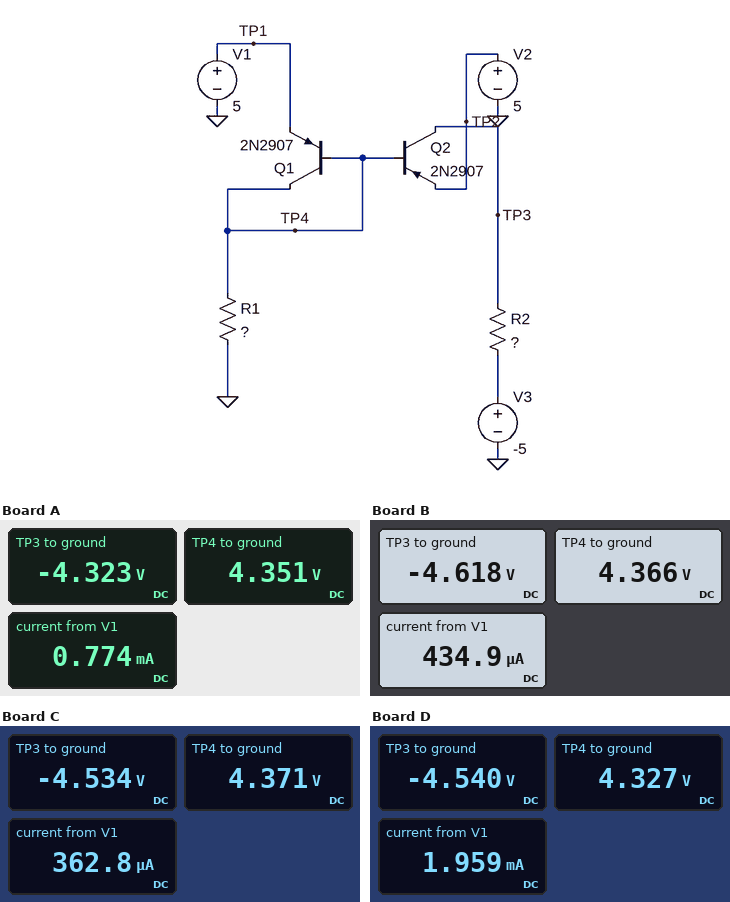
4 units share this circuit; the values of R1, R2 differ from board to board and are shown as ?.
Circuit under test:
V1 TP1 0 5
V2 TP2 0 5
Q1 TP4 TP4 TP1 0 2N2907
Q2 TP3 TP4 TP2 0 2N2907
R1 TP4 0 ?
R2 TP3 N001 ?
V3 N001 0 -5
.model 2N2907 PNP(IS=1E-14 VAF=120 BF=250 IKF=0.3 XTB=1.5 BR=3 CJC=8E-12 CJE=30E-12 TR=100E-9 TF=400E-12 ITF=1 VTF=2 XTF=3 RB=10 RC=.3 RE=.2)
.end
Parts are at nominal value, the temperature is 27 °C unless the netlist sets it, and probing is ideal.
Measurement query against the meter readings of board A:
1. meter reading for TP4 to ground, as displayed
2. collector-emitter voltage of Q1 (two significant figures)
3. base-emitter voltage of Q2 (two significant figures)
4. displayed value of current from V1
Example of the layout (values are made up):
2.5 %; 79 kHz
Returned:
4.351 V; -650 mV; -650 mV; 0.774 mA
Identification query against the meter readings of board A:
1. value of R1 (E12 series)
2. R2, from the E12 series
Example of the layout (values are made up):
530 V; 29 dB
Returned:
5.6 kΩ; 820 Ω
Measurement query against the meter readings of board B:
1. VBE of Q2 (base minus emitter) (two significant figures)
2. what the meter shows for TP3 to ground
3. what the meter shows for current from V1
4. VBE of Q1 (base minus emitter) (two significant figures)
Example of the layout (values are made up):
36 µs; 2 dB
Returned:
-630 mV; -4.618 V; 434.9 µA; -630 mV
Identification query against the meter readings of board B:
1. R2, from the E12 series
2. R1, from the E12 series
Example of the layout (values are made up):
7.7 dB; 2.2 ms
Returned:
820 Ω; 10 kΩ
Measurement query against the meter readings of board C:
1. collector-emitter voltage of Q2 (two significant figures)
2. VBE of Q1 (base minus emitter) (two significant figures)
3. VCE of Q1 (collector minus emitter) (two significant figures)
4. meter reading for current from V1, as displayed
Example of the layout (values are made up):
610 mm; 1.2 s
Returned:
-9.5 V; -630 mV; -630 mV; 362.8 µA
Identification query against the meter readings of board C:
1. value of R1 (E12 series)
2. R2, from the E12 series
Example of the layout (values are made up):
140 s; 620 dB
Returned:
12 kΩ; 1.2 kΩ
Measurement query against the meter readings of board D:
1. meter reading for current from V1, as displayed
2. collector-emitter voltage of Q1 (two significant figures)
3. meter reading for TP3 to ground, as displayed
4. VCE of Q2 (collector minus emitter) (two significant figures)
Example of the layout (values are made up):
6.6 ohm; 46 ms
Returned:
1.959 mA; -670 mV; -4.540 V; -9.5 V
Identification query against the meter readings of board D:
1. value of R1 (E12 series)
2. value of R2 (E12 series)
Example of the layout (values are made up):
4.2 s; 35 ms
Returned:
2.2 kΩ; 220 Ω
